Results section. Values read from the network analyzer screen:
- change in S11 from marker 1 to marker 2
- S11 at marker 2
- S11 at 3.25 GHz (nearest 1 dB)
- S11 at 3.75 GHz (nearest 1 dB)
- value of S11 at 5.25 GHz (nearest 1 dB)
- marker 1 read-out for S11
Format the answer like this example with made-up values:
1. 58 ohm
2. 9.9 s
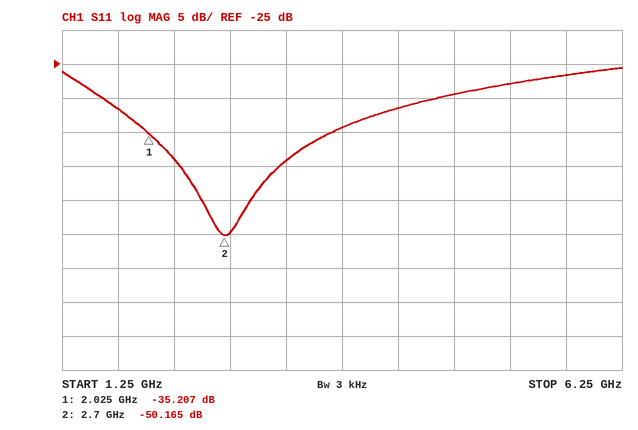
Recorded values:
1. -14.958 dB
2. -50.165 dB
3. -39 dB
4. -34 dB
5. -28 dB
6. -35.207 dB
